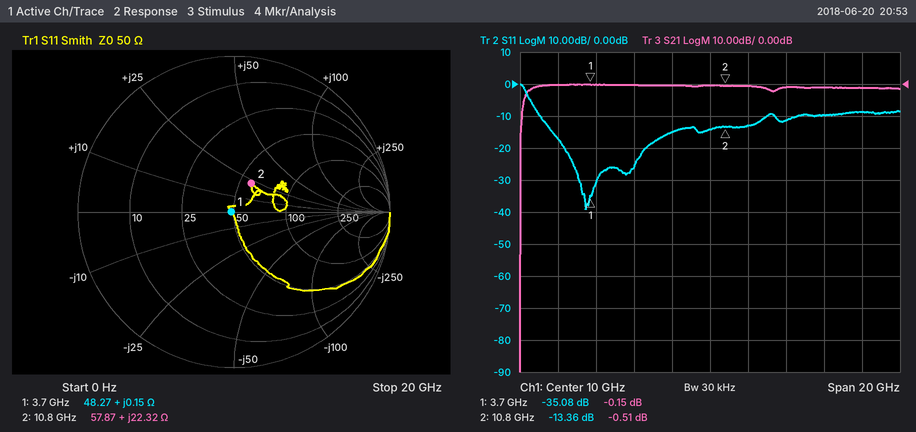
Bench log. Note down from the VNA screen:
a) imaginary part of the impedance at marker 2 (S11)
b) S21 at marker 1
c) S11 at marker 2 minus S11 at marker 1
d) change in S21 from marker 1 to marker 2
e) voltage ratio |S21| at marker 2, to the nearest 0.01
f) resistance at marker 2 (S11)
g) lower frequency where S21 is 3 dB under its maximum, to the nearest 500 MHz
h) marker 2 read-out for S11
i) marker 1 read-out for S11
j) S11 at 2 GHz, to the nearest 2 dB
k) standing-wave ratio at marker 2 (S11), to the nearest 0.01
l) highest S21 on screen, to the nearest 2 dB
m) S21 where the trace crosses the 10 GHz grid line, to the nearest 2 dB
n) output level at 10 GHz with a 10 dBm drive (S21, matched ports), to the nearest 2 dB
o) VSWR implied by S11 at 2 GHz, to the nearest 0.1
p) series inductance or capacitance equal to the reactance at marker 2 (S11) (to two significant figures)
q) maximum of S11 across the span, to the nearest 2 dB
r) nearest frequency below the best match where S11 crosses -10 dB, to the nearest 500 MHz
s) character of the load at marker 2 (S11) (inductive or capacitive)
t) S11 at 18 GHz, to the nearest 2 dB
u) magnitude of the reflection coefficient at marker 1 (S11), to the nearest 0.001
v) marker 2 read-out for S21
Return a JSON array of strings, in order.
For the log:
["+22.32 Ω", "-0.15 dB", "21.72 dB", "-0.36 dB", "0.94", "57.87 Ω", "500 MHz", "-13.36 dB", "-35.08 dB", "-18 dB", "1.55", "0 dB", "0 dB", "10 dBm", "1.3", "330 pH", "0 dB", "1.0 GHz", "inductive", "-8 dB", "0.018", "-0.51 dB"]
